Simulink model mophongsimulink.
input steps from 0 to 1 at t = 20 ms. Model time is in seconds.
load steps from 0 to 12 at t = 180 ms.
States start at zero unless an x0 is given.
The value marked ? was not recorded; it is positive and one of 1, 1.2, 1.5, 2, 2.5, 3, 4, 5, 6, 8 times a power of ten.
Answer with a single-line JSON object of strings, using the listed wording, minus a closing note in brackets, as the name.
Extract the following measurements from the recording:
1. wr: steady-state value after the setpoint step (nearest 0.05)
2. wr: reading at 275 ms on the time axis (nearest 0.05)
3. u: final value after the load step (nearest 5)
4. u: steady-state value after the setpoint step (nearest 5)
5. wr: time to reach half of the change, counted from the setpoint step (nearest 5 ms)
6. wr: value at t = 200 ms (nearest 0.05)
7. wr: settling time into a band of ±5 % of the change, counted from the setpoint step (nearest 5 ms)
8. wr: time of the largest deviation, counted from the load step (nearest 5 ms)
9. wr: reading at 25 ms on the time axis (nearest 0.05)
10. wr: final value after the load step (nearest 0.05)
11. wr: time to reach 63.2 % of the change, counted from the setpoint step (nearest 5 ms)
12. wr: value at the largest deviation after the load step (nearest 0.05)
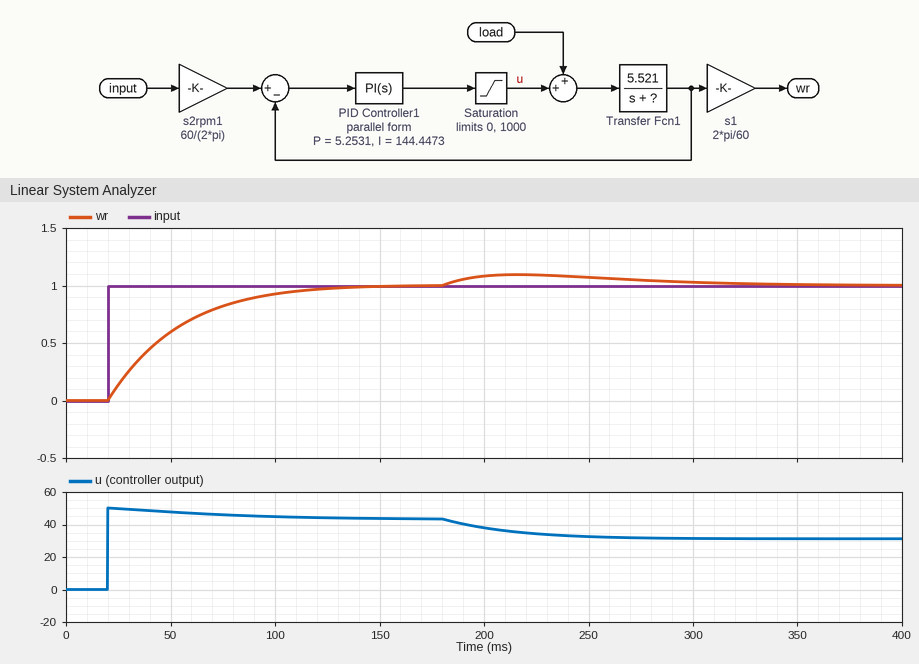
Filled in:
{"wr: steady-state value after the setpoint step": "1.00", "wr: reading at 275 ms on the time axis": "1.05", "u: final value after the load step": "30", "u: steady-state value after the setpoint step": "45", "wr: time to reach half of the change, counted from the setpoint step": "25 ms", "wr: value at t = 200 ms": "1.10", "wr: settling time into a band of ±5 % of the change, counted from the setpoint step": "90 ms", "wr: time of the largest deviation, counted from the load step": "35 ms", "wr: reading at 25 ms on the time axis": "0.15", "wr: final value after the load step": "1.00", "wr: time to reach 63.2 % of the change, counted from the setpoint step": "35 ms", "wr: value at the largest deviation after the load step": "1.10"}
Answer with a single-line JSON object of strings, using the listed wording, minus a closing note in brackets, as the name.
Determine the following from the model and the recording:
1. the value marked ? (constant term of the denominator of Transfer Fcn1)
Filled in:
{"the value marked ?": "25"}
